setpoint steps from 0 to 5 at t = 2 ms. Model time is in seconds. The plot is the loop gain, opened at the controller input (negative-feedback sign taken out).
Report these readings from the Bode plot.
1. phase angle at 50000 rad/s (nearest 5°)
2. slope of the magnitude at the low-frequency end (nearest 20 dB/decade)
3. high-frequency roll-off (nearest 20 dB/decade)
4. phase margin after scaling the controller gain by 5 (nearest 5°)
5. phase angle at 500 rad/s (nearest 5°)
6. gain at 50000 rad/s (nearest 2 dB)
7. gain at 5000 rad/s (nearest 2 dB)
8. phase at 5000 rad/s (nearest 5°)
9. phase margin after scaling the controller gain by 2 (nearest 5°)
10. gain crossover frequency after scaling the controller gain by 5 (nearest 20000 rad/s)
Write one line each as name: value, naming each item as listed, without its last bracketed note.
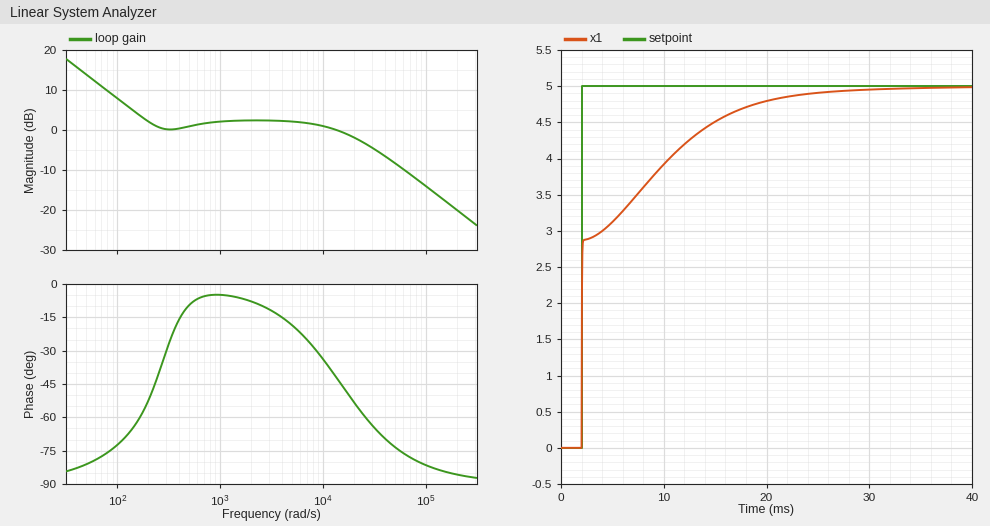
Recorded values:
phase angle at 50000 rad/s: -75°
slope of the magnitude at the low-frequency end: -20 dB/decade
high-frequency roll-off: -20 dB/decade
phase margin after scaling the controller gain by 5: 100°
phase angle at 500 rad/s: -10°
gain at 50000 rad/s: -8 dB
gain at 5000 rad/s: 2 dB
phase at 5000 rad/s: -20°
phase margin after scaling the controller gain by 2: 110°
gain crossover frequency after scaling the controller gain by 5: 100000 rad/s
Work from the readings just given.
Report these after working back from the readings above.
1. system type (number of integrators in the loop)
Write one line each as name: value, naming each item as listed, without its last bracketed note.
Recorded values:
system type: 1
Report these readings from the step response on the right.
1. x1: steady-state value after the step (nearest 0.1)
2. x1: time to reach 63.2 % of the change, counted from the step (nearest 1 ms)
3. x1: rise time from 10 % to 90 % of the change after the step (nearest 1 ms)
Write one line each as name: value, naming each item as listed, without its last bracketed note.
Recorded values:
x1: steady-state value after the step: 5.0
x1: time to reach 63.2 % of the change, counted from the step: 3 ms
x1: rise time from 10 % to 90 % of the change after the step: 13 ms
